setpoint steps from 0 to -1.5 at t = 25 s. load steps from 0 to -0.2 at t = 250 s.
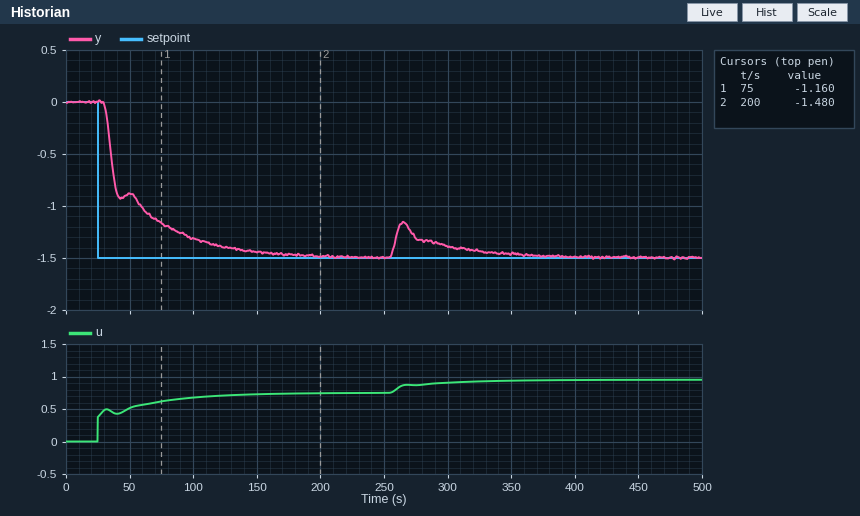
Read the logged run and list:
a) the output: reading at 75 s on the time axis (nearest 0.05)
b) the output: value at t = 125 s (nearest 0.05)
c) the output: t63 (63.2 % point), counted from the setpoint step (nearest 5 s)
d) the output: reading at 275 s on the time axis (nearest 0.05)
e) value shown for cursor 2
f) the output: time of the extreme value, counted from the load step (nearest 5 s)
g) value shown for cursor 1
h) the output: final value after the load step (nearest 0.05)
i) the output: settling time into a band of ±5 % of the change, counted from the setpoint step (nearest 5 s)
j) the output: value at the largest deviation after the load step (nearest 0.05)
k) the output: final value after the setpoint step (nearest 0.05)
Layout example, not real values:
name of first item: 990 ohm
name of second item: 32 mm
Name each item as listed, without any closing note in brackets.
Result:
the output: reading at 75 s on the time axis: -1.15
the output: value at t = 125 s: -1.40
the output: t63 (63.2 % point), counted from the setpoint step: 30 s
the output: reading at 275 s on the time axis: -1.30
value shown for cursor 2: -1.480
the output: time of the extreme value, counted from the load step: 15 s
value shown for cursor 1: -1.160
the output: final value after the load step: -1.50
the output: settling time into a band of ±5 % of the change, counted from the setpoint step: 115 s
the output: value at the largest deviation after the load step: -1.15
the output: final value after the setpoint step: -1.50
